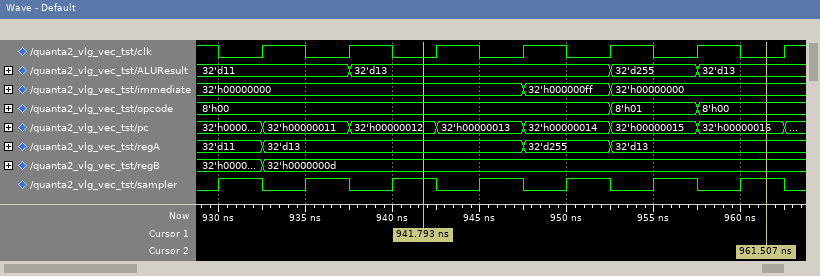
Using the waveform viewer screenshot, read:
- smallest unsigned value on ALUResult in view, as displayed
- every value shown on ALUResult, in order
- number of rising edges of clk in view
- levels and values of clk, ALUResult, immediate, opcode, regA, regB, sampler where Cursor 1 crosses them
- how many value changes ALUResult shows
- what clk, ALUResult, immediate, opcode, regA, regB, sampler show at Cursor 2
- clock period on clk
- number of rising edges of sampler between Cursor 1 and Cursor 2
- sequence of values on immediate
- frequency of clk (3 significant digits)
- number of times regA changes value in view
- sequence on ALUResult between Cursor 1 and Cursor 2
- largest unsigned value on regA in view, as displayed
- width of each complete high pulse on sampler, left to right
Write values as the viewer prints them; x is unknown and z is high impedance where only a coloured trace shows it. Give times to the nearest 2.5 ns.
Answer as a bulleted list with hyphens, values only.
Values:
- 32'd11
- 32'd11, 32'd13, 32'd255, 32'd13
- 7
- clk=0, ALUResult=32'd13, immediate=32'h00000000, opcode=8'h00, regA=32'd13, regB=32'h0000000d, sampler=1
- 3
- clk=0, ALUResult=32'd13, immediate=32'h00000000, opcode=8'h00, regA=32'd13, regB=32'h0000000d, sampler=1
- 5 ns
- 4
- 32'h00000000, 32'h000000ff, 32'h00000000
- 200 MHz
- 3
- 32'd13, 32'd255, 32'd13
- 32'd255
- 2.5 ns, 2.5 ns, 2.5 ns, 2.5 ns, 2.5 ns, 2.5 ns, 2.5 ns
